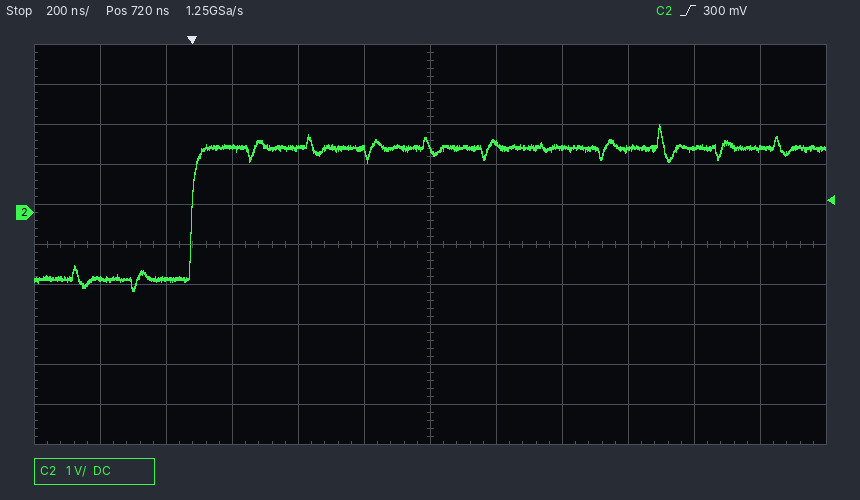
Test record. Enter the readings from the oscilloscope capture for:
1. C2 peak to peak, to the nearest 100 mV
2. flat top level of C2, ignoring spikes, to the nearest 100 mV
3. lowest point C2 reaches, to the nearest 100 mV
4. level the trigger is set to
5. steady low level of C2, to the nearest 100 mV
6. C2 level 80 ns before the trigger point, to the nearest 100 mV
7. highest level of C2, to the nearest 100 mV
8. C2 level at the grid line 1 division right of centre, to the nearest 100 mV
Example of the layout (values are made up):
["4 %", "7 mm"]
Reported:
["4.2 V", "1.6 V", "-2.0 V", "300 mV", "-1.7 V", "-1.7 V", "2.2 V", "1.7 V"]
